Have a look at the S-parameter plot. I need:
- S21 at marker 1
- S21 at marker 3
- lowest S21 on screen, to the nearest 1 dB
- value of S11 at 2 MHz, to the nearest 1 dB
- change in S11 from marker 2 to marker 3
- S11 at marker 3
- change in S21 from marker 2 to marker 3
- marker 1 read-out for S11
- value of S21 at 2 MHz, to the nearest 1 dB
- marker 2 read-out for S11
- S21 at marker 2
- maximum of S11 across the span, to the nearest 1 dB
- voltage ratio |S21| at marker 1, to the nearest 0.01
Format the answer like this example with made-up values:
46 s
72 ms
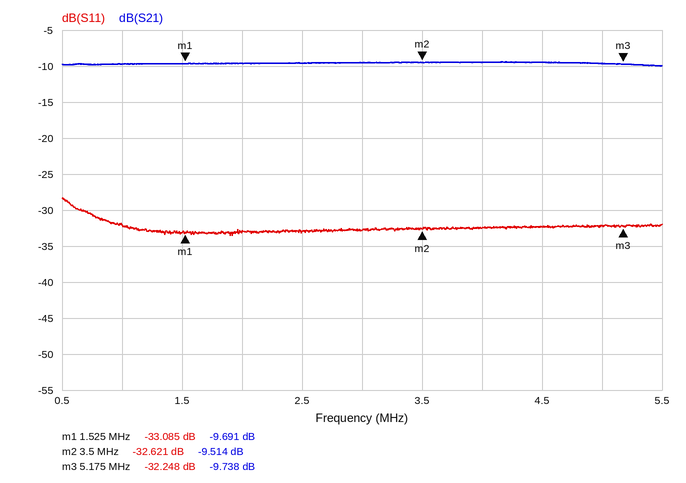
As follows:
-9.691 dB
-9.738 dB
-10 dB
-33 dB
0.373 dB
-32.248 dB
-0.224 dB
-33.085 dB
-10 dB
-32.621 dB
-9.514 dB
-28 dB
0.33
